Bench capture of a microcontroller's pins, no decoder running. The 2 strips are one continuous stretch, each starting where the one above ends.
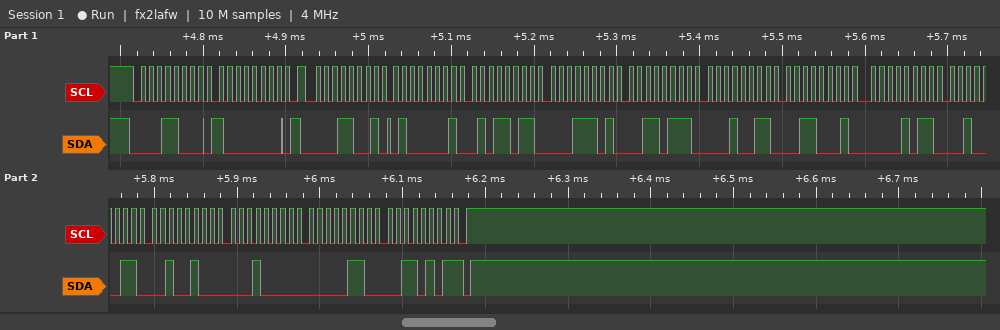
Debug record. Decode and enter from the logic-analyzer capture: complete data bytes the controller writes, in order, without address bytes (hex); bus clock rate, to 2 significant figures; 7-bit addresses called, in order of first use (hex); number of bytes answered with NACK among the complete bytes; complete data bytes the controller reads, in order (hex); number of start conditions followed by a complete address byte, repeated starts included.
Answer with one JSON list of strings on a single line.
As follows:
["80", "100 kHz", "0x0C", "1", "41 5B 1D 37 13 31 0B 23 24 10 06 35", "2"]
